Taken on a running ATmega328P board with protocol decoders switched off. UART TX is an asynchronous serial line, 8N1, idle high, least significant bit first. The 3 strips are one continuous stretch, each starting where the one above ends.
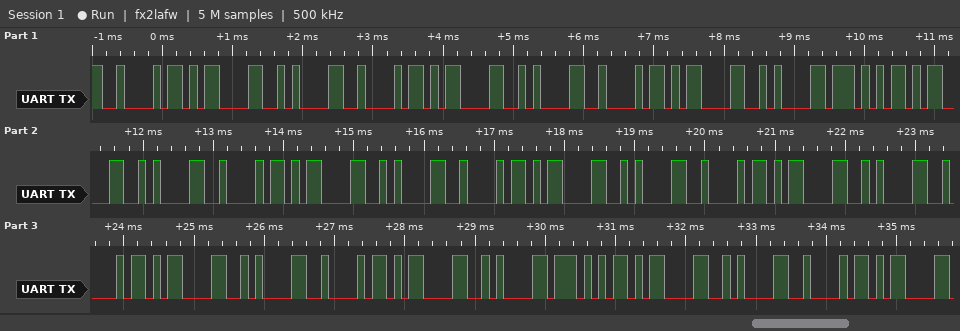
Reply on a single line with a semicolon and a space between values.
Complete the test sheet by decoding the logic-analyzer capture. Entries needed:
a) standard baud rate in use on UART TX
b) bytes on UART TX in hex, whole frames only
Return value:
9600 baud; 0x42 0x0D 0x0A 0x42 0x0D 0x0A 0x42 0x0D 0x0A 0x57 0x0D 0x0A 0x42 0x0D 0x0A 0x42 0x0D 0x0A 0x42 0x0D 0x0A 0x42 0x0D 0x0A 0x42 0x0D 0x0A 0x57 0x0D 0x0A 0x42 0x0D
